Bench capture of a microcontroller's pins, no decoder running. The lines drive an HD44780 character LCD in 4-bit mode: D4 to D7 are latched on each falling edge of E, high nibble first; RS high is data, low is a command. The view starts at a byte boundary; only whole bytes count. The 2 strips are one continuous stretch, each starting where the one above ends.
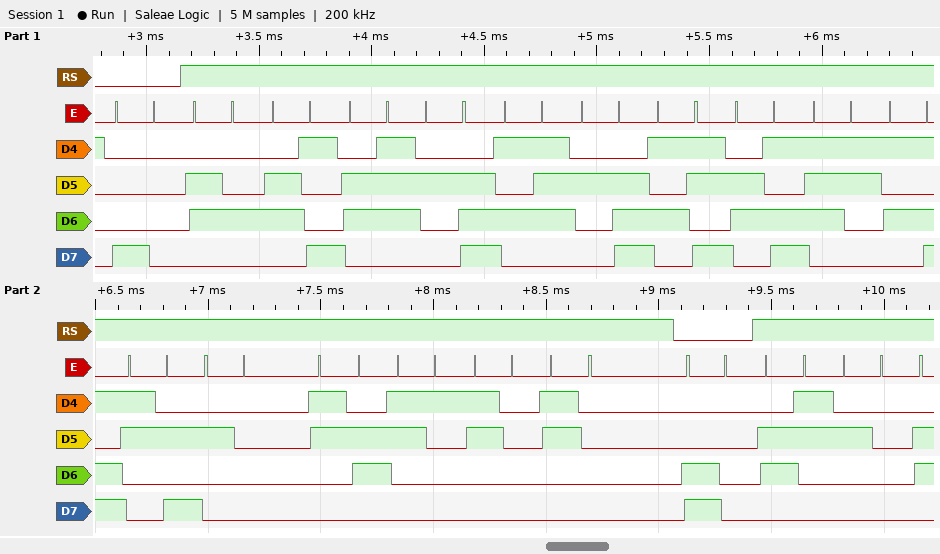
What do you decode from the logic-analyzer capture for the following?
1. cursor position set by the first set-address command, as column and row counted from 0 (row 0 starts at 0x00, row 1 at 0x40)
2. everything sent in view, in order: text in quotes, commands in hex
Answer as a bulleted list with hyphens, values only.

- column 0, row 0
- 0x80 "dig.W.[ms]: 6100" 0xC0 "c "
